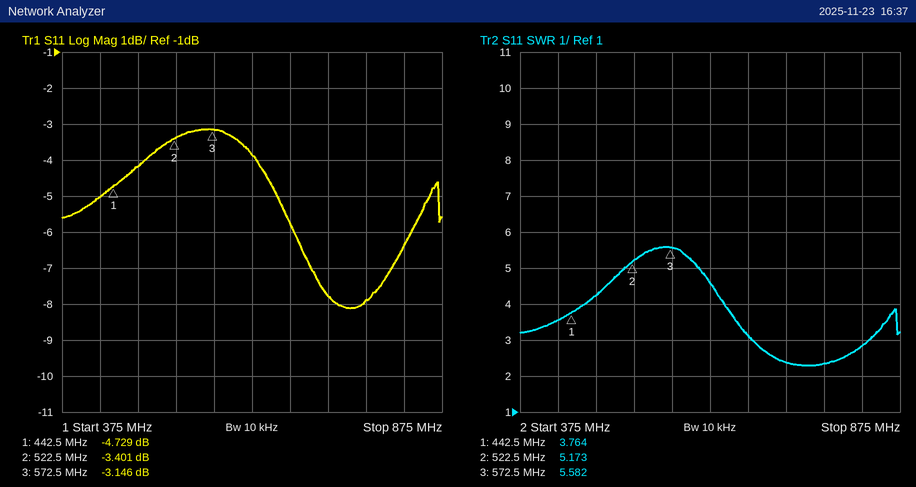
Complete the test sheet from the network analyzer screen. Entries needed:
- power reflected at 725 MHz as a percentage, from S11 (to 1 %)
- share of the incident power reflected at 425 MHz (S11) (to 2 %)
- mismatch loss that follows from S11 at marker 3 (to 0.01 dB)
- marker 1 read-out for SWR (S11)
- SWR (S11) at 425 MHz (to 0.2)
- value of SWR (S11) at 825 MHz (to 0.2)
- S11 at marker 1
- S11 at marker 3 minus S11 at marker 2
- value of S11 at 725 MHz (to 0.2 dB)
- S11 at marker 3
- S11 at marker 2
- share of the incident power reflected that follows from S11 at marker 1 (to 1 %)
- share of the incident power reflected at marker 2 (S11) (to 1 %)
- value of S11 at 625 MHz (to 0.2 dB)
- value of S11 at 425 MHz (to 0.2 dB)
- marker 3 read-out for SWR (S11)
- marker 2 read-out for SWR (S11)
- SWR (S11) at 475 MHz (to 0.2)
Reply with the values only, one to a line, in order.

17 %
32 %
2.88 dB
3.764
3.6
2.8
-4.729 dB
0.255 dB
-7.8 dB
-3.146 dB
-3.401 dB
34 %
46 %
-3.8 dB
-5.0 dB
5.582
5.173
4.2
